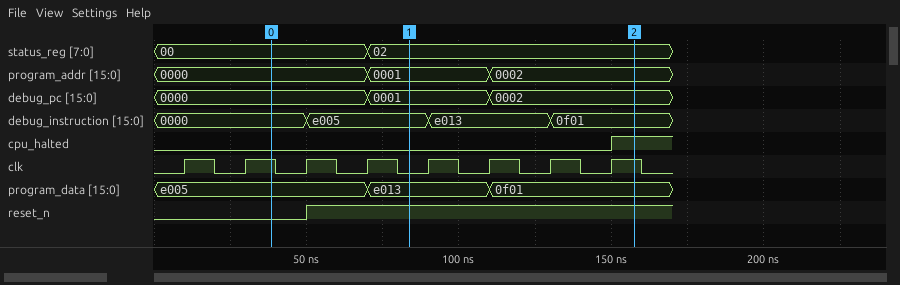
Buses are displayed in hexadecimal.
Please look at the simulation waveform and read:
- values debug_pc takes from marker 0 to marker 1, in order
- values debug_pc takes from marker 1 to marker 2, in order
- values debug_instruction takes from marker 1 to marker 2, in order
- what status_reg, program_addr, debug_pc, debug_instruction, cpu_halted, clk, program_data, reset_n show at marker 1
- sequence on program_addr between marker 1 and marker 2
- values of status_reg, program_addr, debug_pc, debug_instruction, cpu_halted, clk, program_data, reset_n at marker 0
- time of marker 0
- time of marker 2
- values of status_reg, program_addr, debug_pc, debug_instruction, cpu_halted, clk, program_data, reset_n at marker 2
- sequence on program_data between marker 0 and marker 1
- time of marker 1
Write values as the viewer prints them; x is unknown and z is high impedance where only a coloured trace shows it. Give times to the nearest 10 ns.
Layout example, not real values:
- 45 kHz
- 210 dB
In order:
- 0000, 0001
- 0001, 0002
- e005, e013, 0f01
- status_reg=02, program_addr=0001, debug_pc=0001, debug_instruction=e005, cpu_halted=0, clk=0, program_data=e013, reset_n=1
- 0001, 0002
- status_reg=00, program_addr=0000, debug_pc=0000, debug_instruction=0000, cpu_halted=0, clk=1, program_data=e005, reset_n=0
- 40 ns
- 160 ns
- status_reg=02, program_addr=0002, debug_pc=0002, debug_instruction=0f01, cpu_halted=1, clk=1, program_data=0f01, reset_n=1
- e005, e013
- 80 ns
